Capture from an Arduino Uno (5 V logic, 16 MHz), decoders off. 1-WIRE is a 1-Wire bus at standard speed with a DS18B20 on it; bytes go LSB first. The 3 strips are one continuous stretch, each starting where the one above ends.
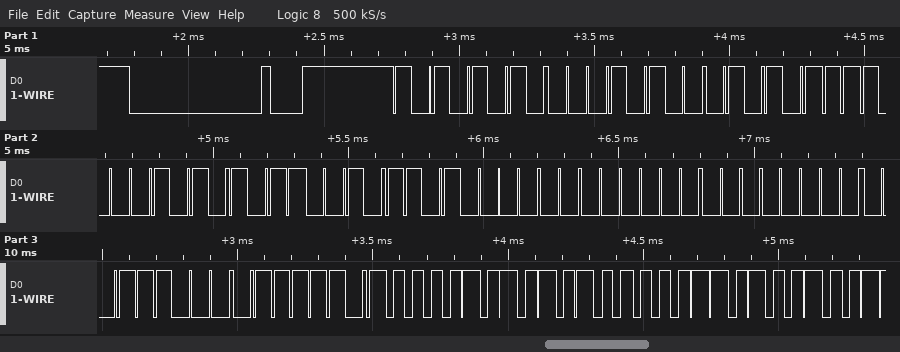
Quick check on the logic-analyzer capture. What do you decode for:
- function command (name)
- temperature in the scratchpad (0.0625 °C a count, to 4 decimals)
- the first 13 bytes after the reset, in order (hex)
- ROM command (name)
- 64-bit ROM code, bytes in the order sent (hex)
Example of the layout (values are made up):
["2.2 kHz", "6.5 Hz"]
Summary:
["Read Scratchpad", "85.0000 °C", "55 28 EA 51 4D 0B 00 00 1C BE 50 05 4B", "Match ROM", "28 EA 51 4D 0B 00 00 1C"]
